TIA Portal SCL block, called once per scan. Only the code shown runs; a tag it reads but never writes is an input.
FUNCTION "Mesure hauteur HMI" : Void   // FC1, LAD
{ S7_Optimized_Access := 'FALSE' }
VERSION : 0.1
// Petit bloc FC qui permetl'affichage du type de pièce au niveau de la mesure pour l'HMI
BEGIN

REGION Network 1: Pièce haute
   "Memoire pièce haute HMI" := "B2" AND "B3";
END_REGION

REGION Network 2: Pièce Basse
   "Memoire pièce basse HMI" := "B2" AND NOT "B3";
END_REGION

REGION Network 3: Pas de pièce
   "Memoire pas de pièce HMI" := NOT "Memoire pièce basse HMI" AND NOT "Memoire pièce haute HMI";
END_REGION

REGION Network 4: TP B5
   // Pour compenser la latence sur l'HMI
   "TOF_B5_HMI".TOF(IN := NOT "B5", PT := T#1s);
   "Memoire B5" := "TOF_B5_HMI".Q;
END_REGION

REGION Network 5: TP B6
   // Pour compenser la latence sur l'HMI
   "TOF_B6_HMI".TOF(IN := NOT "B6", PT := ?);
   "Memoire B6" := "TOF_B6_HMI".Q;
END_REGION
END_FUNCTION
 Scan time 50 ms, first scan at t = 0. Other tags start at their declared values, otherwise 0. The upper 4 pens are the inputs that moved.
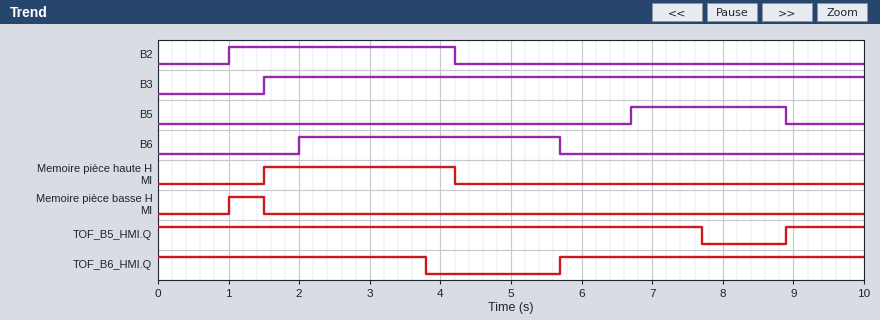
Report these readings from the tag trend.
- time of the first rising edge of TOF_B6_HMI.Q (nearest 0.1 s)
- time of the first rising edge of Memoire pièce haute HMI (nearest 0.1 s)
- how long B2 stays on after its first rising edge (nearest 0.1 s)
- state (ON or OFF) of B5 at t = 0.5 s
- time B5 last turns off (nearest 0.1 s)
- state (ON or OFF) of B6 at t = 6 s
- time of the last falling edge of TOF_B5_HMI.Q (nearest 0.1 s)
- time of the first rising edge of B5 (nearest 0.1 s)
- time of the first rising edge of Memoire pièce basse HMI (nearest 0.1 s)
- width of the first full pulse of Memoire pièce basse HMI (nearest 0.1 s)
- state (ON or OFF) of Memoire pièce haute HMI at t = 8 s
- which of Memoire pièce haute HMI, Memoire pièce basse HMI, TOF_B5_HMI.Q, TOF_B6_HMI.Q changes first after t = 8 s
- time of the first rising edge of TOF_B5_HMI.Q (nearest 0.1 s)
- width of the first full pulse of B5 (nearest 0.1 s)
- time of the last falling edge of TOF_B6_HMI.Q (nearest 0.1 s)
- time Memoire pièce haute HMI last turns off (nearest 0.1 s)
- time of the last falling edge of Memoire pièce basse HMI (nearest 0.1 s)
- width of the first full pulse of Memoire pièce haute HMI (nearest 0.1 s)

5.7 s
1.5 s
3.2 s
OFF
8.9 s
OFF
7.7 s
6.7 s
1.0 s
0.5 s
OFF
TOF_B5_HMI.Q
8.9 s
2.2 s
3.8 s
4.2 s
1.5 s
2.7 s
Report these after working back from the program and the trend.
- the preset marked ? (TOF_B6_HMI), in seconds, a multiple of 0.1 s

1.8 s
